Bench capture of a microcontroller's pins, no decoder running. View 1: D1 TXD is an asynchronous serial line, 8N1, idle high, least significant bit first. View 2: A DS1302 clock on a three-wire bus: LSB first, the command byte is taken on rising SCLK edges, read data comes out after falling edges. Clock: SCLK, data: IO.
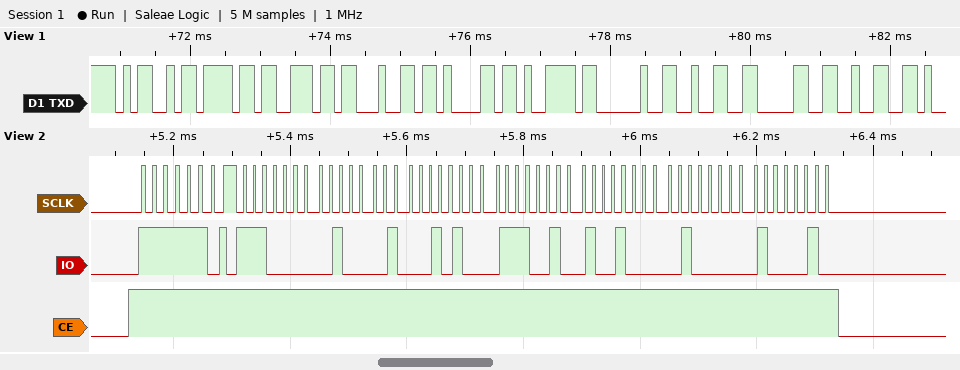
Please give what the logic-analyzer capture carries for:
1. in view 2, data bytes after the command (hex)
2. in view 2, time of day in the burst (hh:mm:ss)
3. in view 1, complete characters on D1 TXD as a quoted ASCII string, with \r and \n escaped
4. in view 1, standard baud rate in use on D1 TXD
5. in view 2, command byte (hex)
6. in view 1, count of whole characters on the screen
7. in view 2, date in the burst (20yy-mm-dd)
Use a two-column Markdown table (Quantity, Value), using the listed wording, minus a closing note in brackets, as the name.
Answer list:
| Quantity | Value |
|---|---|
| in view 2, data bytes after the command | 07 42 14 27 09 02 21 |
| in view 2, time of day in the burst | 14:42:07 |
| in view 1, complete characters on D1 TXD as a quoted ASCII string, with \r and \n escaped | "Monday 202" |
| in view 1, standard baud rate in use on D1 TXD | 9600 baud |
| in view 2, command byte | 0xBF |
| in view 1, count of whole characters on the screen | 10 |
| in view 2, date in the burst | 2021-09-27 |
